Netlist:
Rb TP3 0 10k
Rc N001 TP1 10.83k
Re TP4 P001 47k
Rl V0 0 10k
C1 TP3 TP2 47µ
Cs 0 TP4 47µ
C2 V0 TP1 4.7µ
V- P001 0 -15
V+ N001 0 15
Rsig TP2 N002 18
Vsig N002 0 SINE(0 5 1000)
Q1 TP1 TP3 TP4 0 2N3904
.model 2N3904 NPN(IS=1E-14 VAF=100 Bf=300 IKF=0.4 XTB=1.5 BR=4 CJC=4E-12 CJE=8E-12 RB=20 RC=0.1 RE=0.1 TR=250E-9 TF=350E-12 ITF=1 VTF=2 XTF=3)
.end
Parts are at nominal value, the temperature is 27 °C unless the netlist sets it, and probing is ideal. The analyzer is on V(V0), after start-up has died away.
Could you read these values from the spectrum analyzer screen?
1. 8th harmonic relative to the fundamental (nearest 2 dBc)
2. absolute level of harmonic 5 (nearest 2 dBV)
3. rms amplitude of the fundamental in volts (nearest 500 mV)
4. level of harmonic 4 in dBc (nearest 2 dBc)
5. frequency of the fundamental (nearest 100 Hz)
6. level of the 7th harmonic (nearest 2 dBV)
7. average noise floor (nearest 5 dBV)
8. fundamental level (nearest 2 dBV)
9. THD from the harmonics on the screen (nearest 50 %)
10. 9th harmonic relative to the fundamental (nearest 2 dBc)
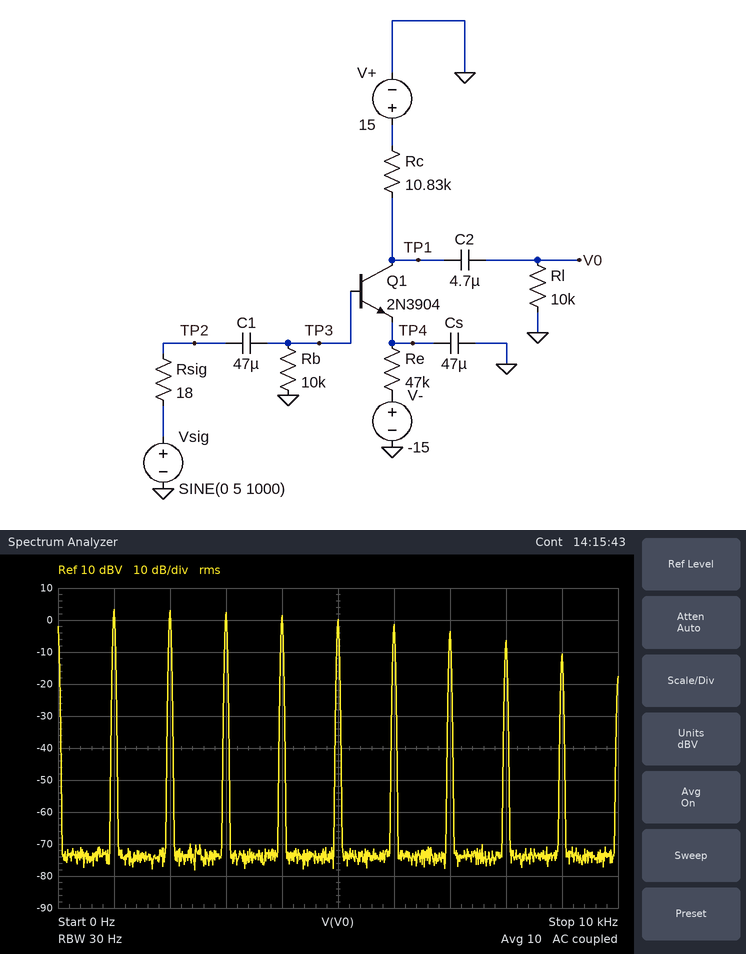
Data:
-10 dBc
0 dBV
1.5 V
-2 dBc
1.0 kHz
-4 dBV
-75 dBV
4 dBV
200 %
-14 dBc
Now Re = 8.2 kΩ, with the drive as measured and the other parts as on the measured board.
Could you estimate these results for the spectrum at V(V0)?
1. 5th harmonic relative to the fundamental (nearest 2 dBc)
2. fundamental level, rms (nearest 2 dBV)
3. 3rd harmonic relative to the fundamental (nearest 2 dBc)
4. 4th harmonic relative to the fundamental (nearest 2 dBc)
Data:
-8 dBc
10 dBV
-2 dBc
-4 dBc
